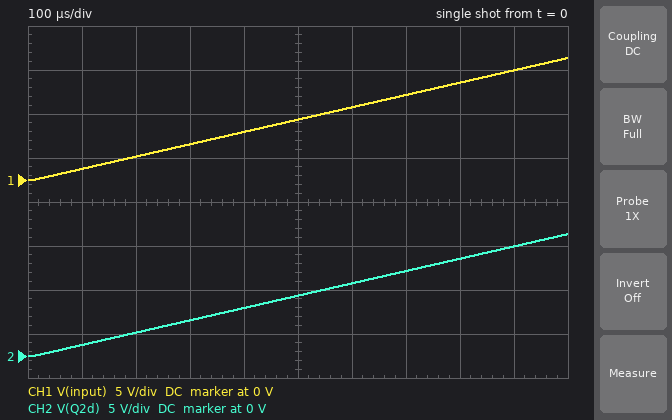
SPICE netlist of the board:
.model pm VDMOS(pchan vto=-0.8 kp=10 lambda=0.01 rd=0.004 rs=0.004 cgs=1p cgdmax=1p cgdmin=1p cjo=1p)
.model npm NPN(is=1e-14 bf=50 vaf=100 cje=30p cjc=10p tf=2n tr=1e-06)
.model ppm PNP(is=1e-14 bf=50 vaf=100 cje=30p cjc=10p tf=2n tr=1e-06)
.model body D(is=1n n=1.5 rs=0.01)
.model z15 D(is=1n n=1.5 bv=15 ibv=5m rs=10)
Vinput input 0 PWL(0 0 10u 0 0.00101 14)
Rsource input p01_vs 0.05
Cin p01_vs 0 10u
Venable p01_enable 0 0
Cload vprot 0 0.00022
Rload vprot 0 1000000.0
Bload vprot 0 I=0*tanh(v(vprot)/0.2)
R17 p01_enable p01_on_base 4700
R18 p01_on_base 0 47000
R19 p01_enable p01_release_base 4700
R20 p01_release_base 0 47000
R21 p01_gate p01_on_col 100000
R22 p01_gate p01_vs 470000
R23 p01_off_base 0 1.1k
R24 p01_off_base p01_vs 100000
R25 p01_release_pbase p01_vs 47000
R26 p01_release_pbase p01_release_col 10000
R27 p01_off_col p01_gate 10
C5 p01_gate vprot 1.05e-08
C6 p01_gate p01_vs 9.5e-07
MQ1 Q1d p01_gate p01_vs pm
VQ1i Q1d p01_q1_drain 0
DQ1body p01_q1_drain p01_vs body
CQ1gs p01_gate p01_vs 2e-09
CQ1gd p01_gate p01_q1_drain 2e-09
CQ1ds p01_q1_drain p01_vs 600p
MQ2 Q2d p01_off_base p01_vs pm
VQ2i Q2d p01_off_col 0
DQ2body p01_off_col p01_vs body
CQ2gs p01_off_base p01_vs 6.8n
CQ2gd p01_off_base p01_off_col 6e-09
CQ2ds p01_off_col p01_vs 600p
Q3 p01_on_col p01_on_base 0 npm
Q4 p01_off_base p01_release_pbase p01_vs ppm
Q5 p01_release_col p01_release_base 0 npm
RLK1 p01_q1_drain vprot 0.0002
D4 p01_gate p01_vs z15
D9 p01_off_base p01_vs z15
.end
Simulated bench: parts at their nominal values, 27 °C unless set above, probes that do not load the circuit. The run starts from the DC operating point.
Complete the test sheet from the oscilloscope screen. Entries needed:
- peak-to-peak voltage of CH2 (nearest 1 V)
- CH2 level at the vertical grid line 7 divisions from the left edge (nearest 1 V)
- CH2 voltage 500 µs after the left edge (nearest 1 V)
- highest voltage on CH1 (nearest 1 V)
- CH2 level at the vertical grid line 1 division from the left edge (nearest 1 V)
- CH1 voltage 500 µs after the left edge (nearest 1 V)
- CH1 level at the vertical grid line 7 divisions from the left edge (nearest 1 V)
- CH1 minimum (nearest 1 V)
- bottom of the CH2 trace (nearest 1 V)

14 V
10 V
7 V
14 V
1 V
7 V
10 V
0 V
0 V
